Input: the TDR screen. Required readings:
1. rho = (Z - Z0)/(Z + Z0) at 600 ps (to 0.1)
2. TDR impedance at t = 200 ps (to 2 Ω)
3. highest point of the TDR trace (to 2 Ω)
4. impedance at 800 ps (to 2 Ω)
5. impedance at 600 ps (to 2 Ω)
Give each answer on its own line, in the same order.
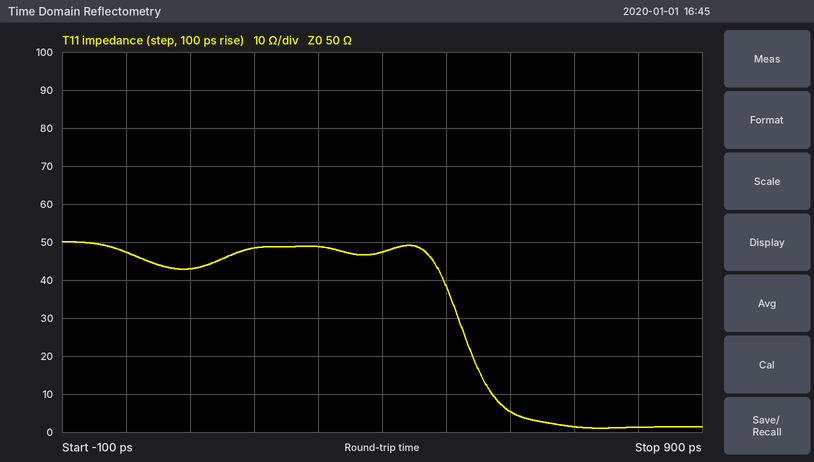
-0.8
48 Ω
50 Ω
2 Ω
6 Ω
